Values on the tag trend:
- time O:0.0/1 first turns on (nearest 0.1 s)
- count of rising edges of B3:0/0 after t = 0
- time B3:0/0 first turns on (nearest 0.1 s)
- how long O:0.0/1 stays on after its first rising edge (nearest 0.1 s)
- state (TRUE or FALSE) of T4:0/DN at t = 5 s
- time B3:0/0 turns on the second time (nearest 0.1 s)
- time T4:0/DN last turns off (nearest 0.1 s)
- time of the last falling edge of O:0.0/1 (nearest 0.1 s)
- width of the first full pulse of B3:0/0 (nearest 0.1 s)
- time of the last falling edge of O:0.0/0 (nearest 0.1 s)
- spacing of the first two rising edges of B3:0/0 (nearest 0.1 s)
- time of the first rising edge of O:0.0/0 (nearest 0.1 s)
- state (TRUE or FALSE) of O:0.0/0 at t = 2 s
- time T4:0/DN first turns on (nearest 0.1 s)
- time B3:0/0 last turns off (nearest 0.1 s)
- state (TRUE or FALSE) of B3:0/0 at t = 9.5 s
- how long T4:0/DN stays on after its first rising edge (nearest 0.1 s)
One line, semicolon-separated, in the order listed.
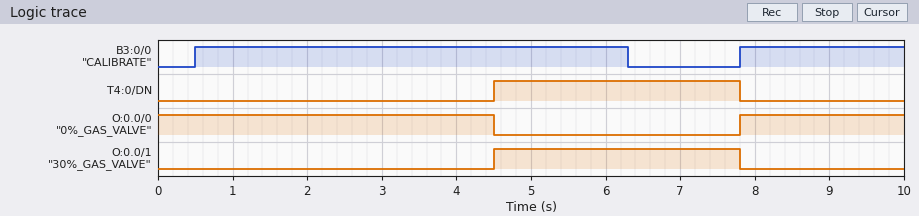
4.5 s; 2; 0.5 s; 3.3 s; TRUE; 7.8 s; 7.8 s; 7.8 s; 5.8 s; 4.5 s; 7.3 s; 7.8 s; TRUE; 4.5 s; 6.3 s; TRUE; 3.3 s
